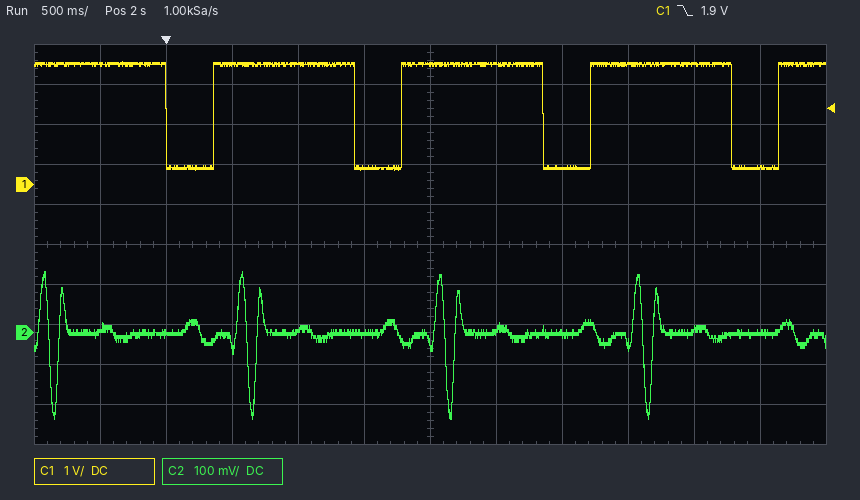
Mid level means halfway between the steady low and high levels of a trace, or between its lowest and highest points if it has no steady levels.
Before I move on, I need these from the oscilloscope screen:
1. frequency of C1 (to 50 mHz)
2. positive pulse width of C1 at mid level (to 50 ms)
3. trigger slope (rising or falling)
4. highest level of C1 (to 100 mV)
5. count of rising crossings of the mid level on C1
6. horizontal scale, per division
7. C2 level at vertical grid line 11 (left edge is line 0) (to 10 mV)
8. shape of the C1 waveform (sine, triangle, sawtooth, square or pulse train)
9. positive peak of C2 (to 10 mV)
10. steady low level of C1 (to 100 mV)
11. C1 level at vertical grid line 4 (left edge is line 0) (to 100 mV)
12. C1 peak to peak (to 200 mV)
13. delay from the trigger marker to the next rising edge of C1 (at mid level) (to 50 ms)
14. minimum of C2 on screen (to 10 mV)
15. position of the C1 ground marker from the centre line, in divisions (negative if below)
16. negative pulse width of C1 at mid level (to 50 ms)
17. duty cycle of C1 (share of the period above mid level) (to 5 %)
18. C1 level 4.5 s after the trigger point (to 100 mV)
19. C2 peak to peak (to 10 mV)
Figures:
700 mHz
1.05 s
falling
3.1 V
4
500 ms
0 mV
pulse train
150 mV
400 mV
3.0 V
2.8 V
350 ms
-220 mV
+1.5 div
350 ms
75 %
400 mV
370 mV
